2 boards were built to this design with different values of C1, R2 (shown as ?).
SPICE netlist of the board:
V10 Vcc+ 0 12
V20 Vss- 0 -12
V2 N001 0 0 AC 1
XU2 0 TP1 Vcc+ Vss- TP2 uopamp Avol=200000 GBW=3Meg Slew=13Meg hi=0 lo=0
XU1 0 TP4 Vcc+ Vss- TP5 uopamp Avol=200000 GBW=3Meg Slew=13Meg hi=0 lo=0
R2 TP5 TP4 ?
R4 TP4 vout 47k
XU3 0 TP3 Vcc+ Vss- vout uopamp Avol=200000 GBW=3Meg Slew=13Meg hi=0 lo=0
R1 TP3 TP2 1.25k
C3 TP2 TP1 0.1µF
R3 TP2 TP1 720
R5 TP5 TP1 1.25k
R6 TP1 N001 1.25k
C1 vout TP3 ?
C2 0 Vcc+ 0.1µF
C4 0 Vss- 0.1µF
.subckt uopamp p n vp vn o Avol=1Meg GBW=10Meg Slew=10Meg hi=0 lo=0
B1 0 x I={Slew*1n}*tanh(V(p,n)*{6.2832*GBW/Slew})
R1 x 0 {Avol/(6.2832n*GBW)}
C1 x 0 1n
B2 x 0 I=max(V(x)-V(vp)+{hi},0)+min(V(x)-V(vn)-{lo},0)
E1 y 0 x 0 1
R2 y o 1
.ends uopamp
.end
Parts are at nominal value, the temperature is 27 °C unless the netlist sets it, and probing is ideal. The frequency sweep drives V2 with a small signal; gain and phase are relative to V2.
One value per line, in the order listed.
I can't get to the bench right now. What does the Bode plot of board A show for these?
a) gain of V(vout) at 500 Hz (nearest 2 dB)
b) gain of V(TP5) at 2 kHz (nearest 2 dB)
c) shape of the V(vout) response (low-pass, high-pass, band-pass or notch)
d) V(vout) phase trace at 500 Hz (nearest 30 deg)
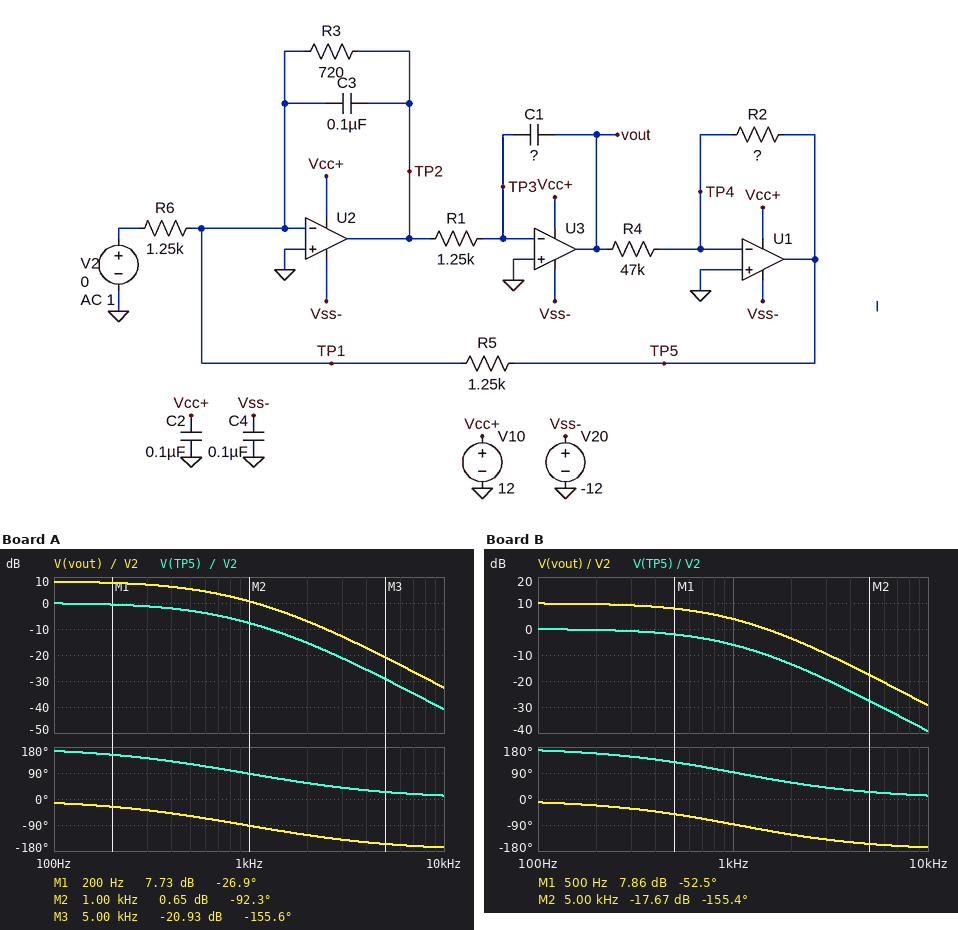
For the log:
6 dB
-16 dB
low-pass
-60 deg
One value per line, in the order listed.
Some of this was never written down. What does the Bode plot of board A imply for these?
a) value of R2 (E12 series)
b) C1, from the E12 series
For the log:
18 kΩ
68 nF
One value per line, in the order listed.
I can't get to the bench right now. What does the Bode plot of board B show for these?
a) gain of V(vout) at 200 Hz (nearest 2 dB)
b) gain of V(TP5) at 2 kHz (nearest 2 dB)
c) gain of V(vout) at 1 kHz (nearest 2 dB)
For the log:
10 dB
-14 dB
4 dB
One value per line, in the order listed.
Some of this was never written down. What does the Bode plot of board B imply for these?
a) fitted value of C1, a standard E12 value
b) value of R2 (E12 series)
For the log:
47 nF
15 kΩ
